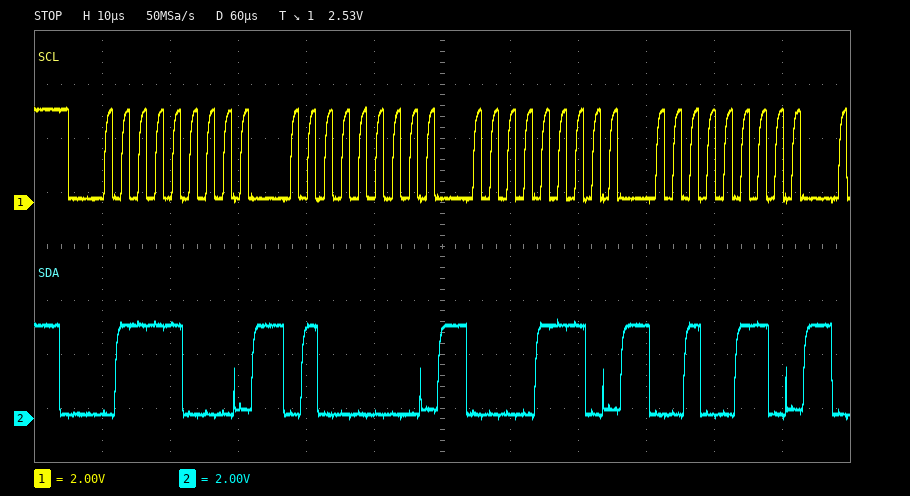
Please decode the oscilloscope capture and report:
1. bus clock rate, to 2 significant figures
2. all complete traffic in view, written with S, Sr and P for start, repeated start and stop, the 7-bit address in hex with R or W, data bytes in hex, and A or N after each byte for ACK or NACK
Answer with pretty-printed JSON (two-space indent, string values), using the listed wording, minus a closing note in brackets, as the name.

{
  "bus clock rate, to 2 significant figures": "400 kHz",
  "all complete traffic in view, written with S, Sr and P for start, repeated start and stop, the 7-bit address in hex with R or W, data bytes in hex, and A or N after each byte for ACK or NACK": "S 3CW A 40 A 0E A 26 A"
}
